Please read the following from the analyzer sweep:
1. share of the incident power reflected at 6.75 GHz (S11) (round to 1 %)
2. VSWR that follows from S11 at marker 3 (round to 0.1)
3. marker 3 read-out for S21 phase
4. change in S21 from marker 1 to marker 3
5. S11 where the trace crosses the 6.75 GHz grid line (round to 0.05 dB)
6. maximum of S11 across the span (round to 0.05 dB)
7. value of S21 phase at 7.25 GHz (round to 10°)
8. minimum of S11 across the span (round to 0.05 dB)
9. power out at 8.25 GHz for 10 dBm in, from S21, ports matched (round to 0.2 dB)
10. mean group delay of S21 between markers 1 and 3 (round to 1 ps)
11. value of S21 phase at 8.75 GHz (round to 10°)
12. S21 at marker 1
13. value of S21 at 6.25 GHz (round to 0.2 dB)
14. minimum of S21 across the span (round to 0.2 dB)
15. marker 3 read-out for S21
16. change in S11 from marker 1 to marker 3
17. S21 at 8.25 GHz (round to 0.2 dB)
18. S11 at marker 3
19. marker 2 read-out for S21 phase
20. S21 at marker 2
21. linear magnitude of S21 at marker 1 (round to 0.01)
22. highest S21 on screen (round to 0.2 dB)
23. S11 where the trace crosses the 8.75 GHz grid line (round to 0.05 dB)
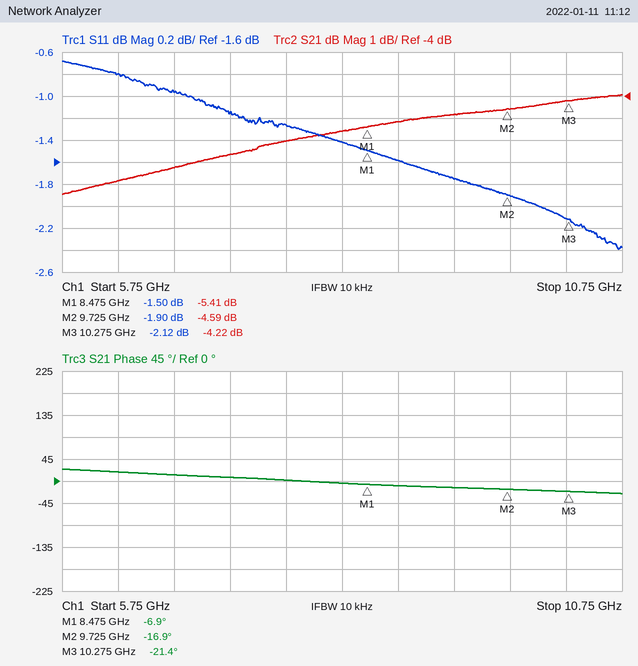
80 %
8.2
-21.4°
1.19 dB
-0.95 dB
-0.70 dB
10°
-2.40 dB
4.4 dBm
22 ps
-10°
-5.41 dB
-7.8 dB
-8.4 dB
-4.22 dB
-0.62 dB
-5.6 dB
-2.12 dB
-16.9°
-4.59 dB
0.54
-4.0 dB
-1.60 dB
